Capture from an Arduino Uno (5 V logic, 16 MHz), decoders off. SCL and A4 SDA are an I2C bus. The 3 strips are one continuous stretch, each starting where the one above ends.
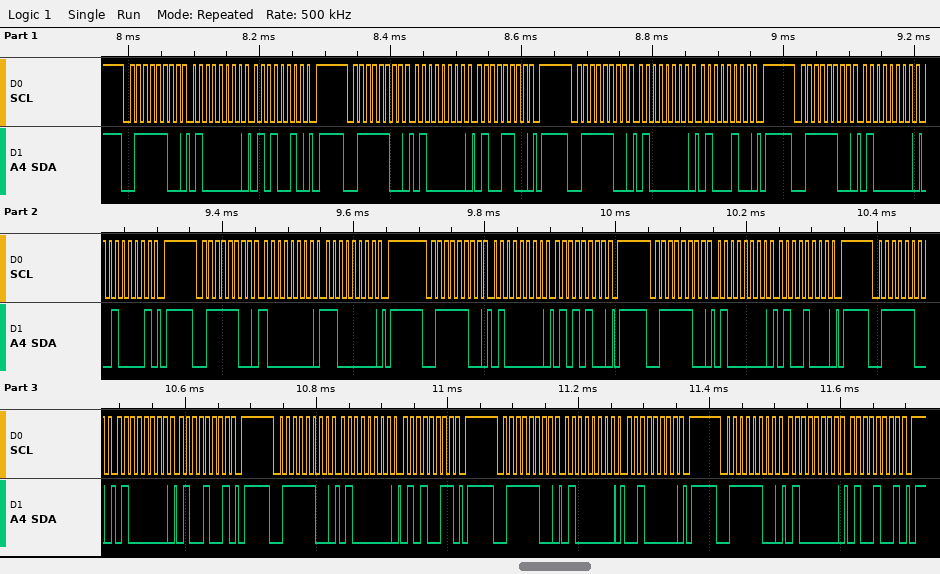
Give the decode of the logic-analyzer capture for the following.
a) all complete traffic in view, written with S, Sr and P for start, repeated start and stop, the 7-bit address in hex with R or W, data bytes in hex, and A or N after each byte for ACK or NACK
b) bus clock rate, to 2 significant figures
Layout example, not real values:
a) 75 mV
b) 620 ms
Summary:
a) S 3EW A 40 A 52 A P S 3EW A 40 A 4C A P S 3EW A 40 A 44 A P S 3EW A 40 A 21 A P S 3EW A 80 A C0 A P S 3EW A 40 A 54 A P S 3EW A 40 A 48 A P S 3EW A 40 A 49 A P S 3EW A 40 A 53 A P S 3EW A 40 A 20 A P S 3EW A 40 A 49 A P
b) 100 kHz
